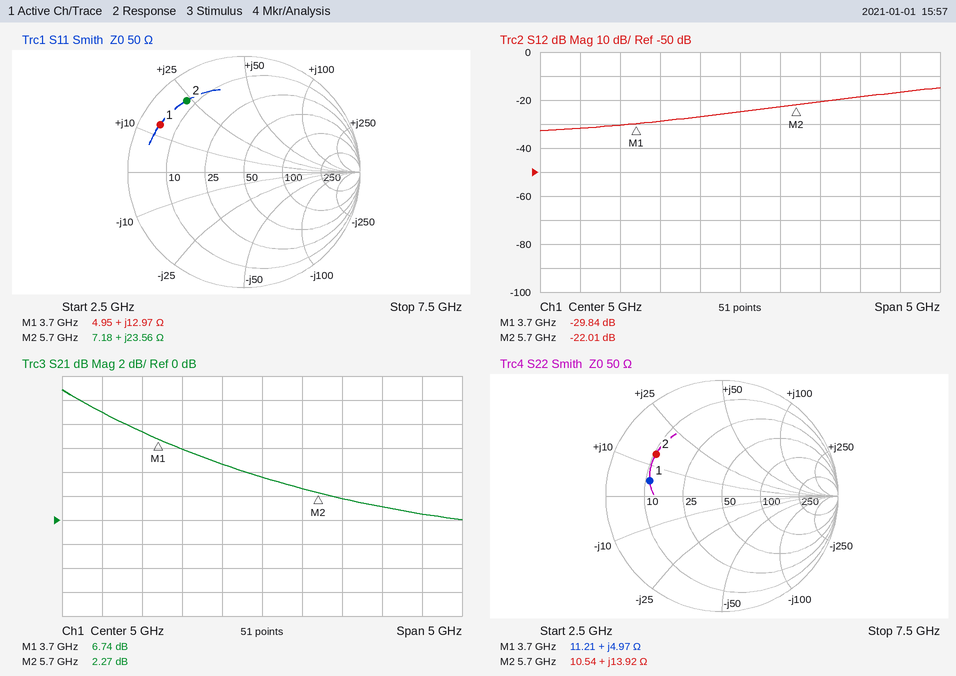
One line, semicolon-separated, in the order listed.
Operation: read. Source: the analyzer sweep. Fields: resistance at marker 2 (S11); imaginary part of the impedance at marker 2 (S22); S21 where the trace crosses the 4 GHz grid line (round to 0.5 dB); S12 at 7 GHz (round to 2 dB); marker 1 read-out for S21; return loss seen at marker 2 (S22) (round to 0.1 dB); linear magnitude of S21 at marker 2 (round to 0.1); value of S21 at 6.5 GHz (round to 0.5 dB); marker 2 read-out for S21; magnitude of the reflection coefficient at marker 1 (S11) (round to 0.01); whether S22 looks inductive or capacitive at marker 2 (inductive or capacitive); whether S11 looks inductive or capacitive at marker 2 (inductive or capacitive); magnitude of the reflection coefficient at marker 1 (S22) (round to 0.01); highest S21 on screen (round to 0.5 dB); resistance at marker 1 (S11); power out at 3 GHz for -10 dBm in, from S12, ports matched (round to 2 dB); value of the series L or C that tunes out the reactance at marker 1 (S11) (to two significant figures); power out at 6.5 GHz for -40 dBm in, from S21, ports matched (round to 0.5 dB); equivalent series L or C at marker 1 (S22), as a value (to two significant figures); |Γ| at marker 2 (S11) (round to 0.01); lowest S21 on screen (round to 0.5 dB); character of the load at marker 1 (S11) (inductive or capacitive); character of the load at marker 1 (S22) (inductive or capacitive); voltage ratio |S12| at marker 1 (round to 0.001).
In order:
7.18 Ω; +13.92 Ω; 6.0 dB; -16 dB; 6.74 dB; 3.4 dB; 1.3; 1.0 dB; 2.27 dB; 0.83; inductive; inductive; 0.64; 11.0 dB; 4.95 Ω; -42 dBm; 3.3 pF; -39.0 dBm; 210 pH; 0.79; 0.0 dB; inductive; inductive; 0.032
